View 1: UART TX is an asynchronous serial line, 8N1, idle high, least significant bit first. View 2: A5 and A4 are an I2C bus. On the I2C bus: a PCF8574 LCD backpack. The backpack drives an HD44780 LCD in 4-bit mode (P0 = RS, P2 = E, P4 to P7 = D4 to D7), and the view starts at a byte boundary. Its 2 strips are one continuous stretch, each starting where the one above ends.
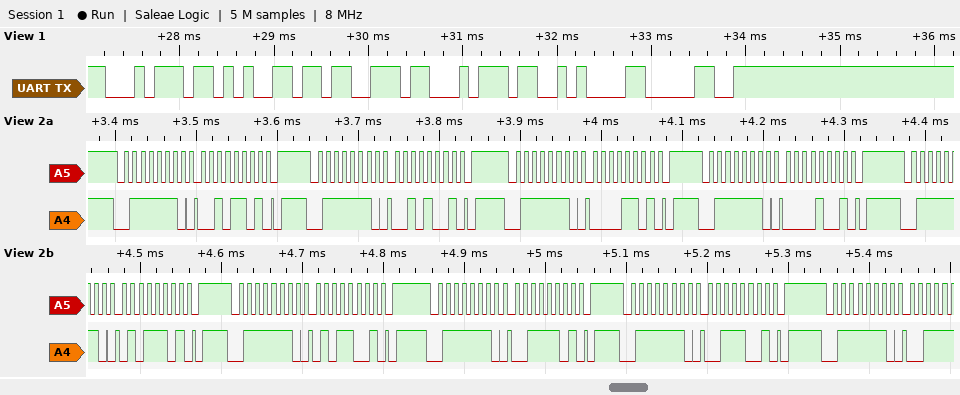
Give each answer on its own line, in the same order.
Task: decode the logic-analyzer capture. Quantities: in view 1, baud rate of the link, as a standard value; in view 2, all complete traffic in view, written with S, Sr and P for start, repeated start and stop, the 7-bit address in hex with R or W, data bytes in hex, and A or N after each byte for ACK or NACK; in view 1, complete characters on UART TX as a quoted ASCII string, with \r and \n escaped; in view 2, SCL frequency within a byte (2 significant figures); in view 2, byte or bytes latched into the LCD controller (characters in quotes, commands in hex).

9600 baud
S 3FW A 2D A P S 3FW A 29 A P S 3FW A 0D A P S 3FW A 09 A P S 3FW A 5D A P S 3FW A 59 A P S 3FW A 3D A P S 3FW A 39 A P S 3FW A
"test\n0"
100 kHz
' ' 'S'
